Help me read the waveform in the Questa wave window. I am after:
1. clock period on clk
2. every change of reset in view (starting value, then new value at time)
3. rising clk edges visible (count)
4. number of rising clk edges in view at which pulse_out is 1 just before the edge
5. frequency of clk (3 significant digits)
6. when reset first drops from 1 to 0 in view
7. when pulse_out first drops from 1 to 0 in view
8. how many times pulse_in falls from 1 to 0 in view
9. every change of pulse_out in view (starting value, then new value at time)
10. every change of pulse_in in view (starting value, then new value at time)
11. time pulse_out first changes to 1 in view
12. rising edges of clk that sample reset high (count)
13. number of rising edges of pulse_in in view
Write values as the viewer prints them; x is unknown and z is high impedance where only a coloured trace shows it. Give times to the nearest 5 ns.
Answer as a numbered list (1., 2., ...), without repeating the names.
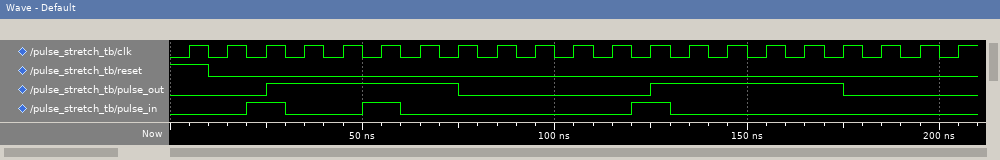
1. 10 ns
2. 1, 0 at 10 ns
3. 21
4. 10
5. 100 MHz
6. 10 ns
7. 75 ns
8. 3
9. 0, 1 at 25 ns, 0 at 75 ns, 1 at 125 ns, 0 at 175 ns
10. 0, 1 at 20 ns, 0 at 30 ns, 1 at 50 ns, 0 at 60 ns, 1 at 120 ns, 0 at 130 ns
11. 25 ns
12. 1
13. 3
